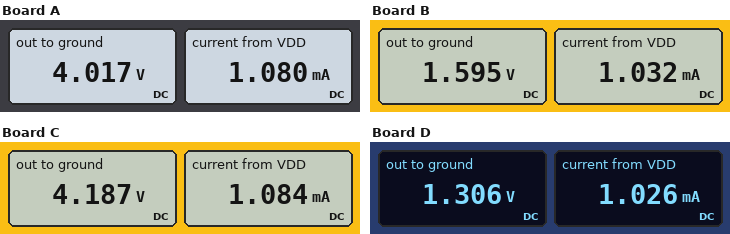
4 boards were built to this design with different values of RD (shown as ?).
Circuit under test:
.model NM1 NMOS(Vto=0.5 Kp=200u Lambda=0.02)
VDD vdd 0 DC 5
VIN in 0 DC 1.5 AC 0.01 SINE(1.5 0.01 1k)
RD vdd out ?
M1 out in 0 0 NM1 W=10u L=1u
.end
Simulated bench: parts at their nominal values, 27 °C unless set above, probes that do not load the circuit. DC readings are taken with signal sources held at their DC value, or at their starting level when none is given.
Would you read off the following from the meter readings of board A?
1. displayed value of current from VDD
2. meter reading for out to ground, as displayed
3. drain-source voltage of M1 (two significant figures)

1.080 mA
4.017 V
4.0 V
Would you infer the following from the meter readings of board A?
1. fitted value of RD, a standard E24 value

910 Ω
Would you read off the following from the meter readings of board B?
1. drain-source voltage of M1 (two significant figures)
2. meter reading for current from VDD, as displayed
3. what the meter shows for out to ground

1.6 V
1.032 mA
1.595 V
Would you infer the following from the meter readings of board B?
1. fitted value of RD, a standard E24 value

3.3 kΩ
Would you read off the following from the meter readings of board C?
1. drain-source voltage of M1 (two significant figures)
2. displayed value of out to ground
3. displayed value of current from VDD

4.2 V
4.187 V
1.084 mA
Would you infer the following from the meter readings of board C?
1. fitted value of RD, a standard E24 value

750 Ω
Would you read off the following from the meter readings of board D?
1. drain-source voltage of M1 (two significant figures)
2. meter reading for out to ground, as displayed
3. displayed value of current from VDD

1.3 V
1.306 V
1.026 mA
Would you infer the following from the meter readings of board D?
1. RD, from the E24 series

3.6 kΩ
